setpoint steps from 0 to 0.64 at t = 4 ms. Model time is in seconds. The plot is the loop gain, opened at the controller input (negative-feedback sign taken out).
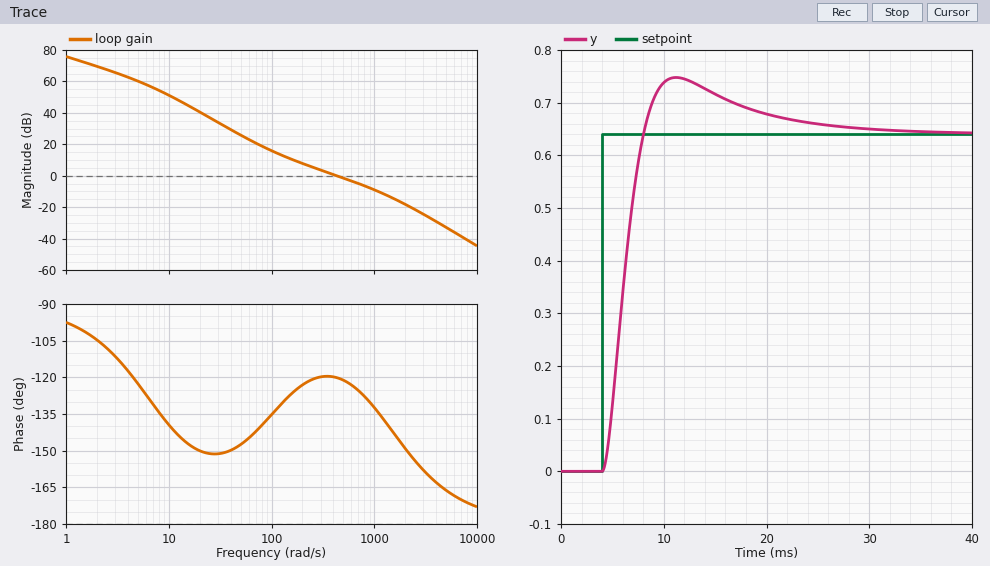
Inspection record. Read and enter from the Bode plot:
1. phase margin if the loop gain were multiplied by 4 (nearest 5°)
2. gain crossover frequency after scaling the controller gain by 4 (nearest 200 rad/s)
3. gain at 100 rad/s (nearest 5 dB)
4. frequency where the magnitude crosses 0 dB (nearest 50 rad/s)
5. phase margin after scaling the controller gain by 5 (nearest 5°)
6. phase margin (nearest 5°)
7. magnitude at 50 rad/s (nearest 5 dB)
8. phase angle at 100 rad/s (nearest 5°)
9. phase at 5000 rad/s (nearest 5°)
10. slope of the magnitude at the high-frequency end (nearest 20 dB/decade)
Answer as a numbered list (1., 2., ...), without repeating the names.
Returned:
1. 40°
2. 1200 rad/s
3. 15 dB
4. 450 rad/s
5. 40°
6. 60°
7. 25 dB
8. -135°
9. -165°
10. -40 dB/decade
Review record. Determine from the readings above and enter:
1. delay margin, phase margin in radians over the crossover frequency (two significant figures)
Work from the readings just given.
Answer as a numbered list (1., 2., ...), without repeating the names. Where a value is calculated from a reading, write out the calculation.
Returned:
1. 60 × π / 180 / 450 = 0.0023 s
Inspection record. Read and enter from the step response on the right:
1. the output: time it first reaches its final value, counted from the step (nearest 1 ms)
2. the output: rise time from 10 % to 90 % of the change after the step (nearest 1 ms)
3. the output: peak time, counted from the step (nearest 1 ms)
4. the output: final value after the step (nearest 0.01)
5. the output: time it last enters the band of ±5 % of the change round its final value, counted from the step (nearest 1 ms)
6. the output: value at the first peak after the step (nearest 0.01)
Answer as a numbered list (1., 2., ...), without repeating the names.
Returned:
1. 4 ms
2. 3 ms
3. 7 ms
4. 0.64
5. 17 ms
6. 0.75
